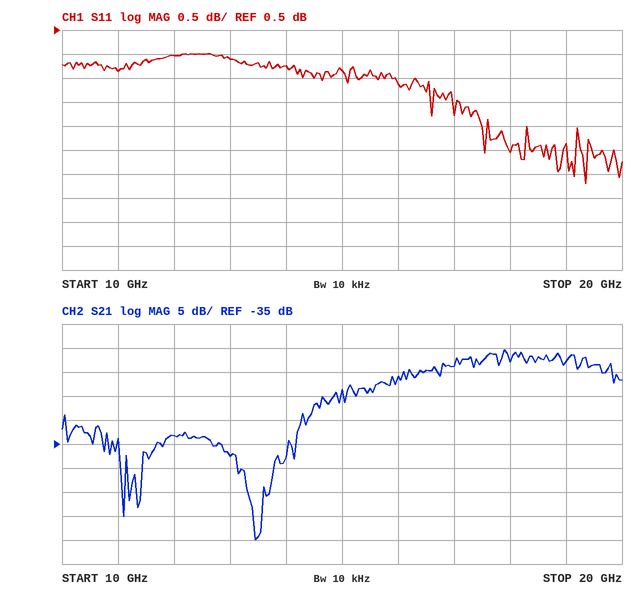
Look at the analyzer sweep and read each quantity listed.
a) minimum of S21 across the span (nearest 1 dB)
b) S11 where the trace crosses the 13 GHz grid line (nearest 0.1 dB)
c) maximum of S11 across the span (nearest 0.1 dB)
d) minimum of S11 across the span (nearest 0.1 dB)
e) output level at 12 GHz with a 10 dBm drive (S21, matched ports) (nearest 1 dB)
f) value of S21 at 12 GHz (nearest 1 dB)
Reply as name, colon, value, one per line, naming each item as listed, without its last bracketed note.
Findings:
minimum of S21 across the span: -55 dB
S11 where the trace crosses the 13 GHz grid line: -0.1 dB
maximum of S11 across the span: 0.0 dB
minimum of S11 across the span: -2.7 dB
output level at 12 GHz with a 10 dBm drive (S21, matched ports): -23 dBm
value of S21 at 12 GHz: -33 dB
